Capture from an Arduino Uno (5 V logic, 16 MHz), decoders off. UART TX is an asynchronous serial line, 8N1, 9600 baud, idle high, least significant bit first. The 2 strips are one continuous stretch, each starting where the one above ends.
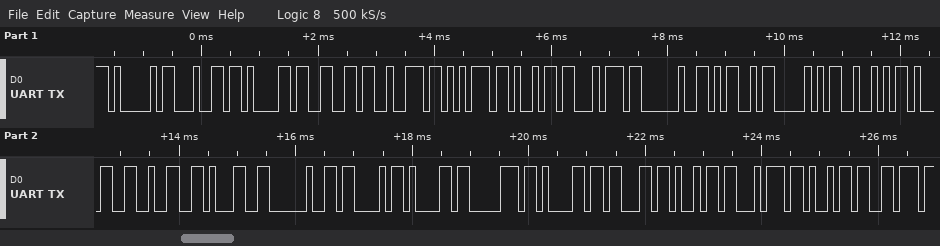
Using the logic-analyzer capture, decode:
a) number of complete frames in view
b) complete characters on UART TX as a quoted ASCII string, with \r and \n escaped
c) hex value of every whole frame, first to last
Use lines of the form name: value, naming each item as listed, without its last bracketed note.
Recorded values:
number of complete frames in view: 25
complete characters on UART TX as a quoted ASCII string, with \r and \n escaped: "Adafruit MPR121 Capacitiv"
hex value of every whole frame, first to last: 41 64 61 66 72 75 69 74 20 4D 50 52 31 32 31 20 43 61 70 61 63 69 74 69 76
